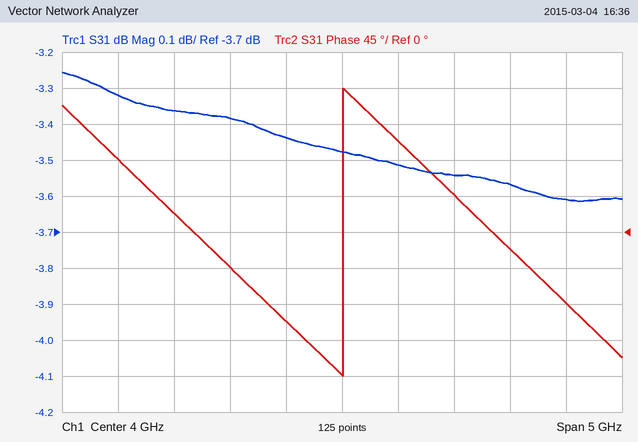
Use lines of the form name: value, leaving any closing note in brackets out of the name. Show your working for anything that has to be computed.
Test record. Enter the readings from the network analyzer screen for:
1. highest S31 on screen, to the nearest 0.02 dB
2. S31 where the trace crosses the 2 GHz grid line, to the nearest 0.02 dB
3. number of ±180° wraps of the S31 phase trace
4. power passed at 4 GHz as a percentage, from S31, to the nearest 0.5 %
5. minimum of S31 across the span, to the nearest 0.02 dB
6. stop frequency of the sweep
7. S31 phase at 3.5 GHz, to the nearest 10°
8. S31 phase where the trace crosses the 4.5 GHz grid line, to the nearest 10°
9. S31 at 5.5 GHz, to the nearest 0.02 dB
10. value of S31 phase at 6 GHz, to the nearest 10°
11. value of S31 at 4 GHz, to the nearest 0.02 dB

highest S31 on screen, to the nearest 0.02 dB: -3.26 dB
S31 where the trace crosses the 2 GHz grid line, to the nearest 0.02 dB: -3.32 dB
number of ±180° wraps of the S31 phase trace: 1
power passed at 4 GHz as a percentage, from S31, to the nearest 0.5 %: 10^(-3.48/10) ≈ 44.9 %, so 45.0 % to the nearest 0.5 %
minimum of S31 across the span, to the nearest 0.02 dB: -3.62 dB
stop frequency of the sweep: 6.5 GHz
S31 phase at 3.5 GHz, to the nearest 10°: -110°
S31 phase where the trace crosses the 4.5 GHz grid line, to the nearest 10°: 110°
S31 at 5.5 GHz, to the nearest 0.02 dB: -3.56 dB
value of S31 phase at 6 GHz, to the nearest 10°: -90°
value of S31 at 4 GHz, to the nearest 0.02 dB: -3.48 dB
